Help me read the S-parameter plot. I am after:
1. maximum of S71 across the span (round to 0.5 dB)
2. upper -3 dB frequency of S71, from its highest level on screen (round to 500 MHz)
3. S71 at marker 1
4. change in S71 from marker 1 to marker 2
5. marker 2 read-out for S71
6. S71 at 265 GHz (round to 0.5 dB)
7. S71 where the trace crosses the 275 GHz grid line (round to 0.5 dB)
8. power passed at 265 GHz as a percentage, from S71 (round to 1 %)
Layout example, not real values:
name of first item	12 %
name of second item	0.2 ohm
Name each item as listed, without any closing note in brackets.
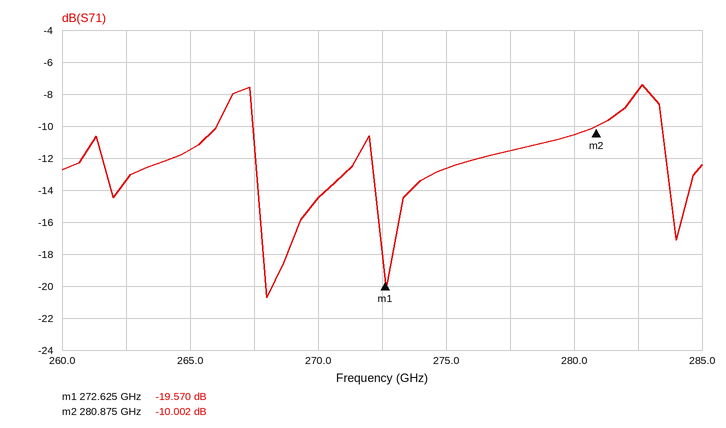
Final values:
maximum of S71 across the span	-7.5 dB
upper -3 dB frequency of S71, from its highest level on screen	283.5 GHz
S71 at marker 1	-19.570 dB
change in S71 from marker 1 to marker 2	9.568 dB
marker 2 read-out for S71	-10.002 dB
S71 at 265 GHz	-11.5 dB
S71 where the trace crosses the 275 GHz grid line	-12.5 dB
power passed at 265 GHz as a percentage, from S71	7 %
